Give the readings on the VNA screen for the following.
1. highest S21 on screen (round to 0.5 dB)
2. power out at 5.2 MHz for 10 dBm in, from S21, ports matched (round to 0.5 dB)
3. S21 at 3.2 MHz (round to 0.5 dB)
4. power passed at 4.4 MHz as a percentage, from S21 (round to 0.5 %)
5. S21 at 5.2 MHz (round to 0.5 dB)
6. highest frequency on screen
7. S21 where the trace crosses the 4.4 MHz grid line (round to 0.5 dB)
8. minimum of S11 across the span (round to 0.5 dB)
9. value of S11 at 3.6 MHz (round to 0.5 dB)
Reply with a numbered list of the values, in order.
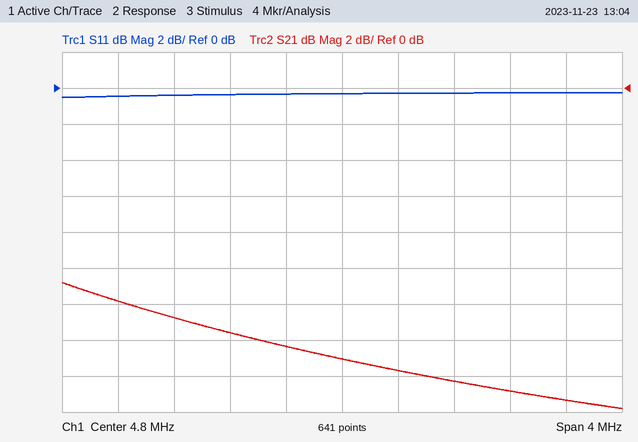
1. -11.0 dB
2. -5.5 dBm
3. -12.0 dB
4. 3.5 %
5. -15.5 dB
6. 6.8 MHz
7. -14.5 dB
8. -0.5 dB
9. -0.5 dB
